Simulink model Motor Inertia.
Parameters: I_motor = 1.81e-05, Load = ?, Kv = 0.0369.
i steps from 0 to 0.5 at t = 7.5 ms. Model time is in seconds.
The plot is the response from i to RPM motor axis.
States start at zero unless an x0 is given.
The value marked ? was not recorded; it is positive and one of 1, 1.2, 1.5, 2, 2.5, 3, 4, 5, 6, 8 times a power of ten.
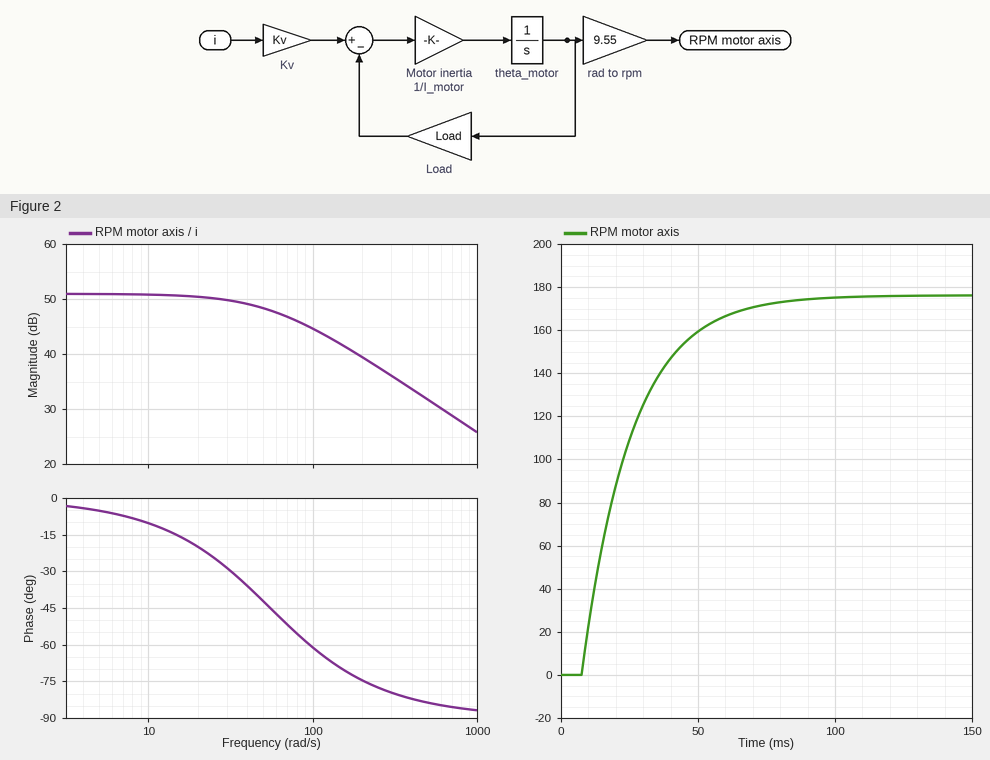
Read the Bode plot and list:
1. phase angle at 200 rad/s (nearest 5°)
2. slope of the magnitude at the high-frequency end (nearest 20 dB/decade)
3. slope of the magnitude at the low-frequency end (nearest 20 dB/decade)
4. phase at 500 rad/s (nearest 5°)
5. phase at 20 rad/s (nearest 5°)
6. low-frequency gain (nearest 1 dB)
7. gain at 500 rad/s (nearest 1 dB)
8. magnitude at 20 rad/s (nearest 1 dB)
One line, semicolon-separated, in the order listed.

-75°; -20 dB/decade; 0 dB/decade; -85°; -20°; 51 dB; 32 dB; 50 dB
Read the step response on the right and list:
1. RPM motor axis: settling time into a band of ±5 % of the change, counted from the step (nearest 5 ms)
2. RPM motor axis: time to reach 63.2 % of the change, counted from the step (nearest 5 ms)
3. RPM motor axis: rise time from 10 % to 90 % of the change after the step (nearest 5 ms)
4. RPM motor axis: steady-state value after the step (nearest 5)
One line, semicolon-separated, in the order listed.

55 ms; 20 ms; 40 ms; 175
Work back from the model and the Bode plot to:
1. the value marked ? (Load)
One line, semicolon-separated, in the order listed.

0.001
